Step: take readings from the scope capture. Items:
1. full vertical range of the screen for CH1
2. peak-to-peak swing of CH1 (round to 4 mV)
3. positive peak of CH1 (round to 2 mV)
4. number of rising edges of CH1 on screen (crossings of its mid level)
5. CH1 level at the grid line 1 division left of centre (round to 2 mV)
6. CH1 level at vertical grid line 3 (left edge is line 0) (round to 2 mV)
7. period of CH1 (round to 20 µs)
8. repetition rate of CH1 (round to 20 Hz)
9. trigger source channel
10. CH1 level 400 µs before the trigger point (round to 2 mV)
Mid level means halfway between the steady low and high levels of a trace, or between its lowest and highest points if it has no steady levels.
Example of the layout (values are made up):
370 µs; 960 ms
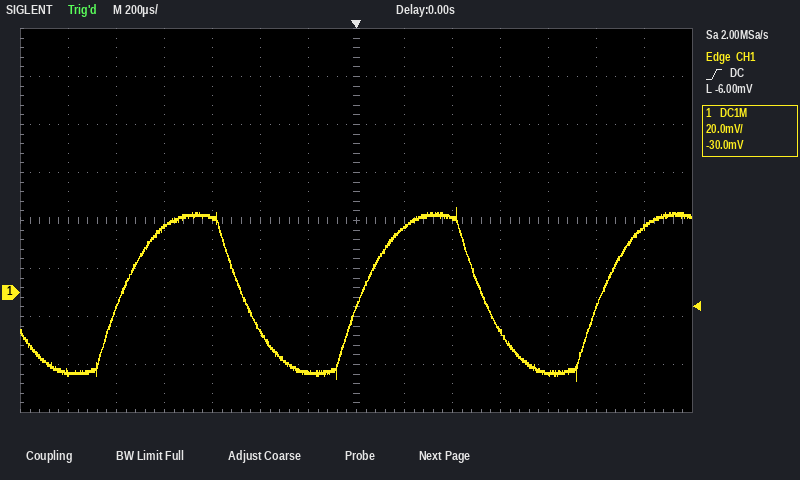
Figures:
160 mV; 72 mV; 36 mV; 3; -34 mV; 28 mV; 1.00 ms; 1.00 kHz; CH1; -16 mV
